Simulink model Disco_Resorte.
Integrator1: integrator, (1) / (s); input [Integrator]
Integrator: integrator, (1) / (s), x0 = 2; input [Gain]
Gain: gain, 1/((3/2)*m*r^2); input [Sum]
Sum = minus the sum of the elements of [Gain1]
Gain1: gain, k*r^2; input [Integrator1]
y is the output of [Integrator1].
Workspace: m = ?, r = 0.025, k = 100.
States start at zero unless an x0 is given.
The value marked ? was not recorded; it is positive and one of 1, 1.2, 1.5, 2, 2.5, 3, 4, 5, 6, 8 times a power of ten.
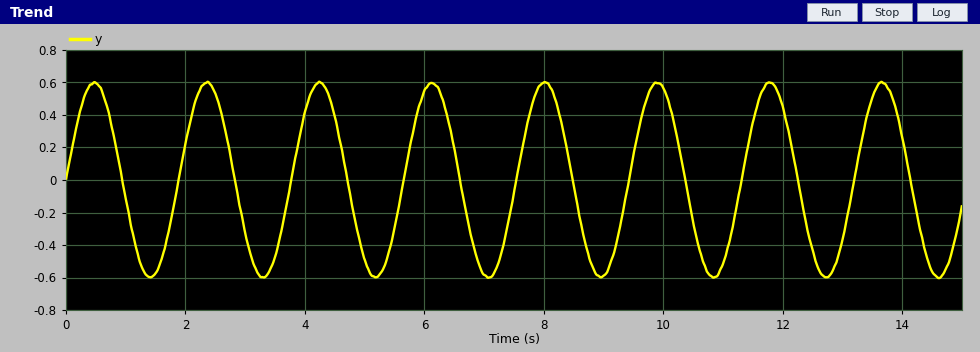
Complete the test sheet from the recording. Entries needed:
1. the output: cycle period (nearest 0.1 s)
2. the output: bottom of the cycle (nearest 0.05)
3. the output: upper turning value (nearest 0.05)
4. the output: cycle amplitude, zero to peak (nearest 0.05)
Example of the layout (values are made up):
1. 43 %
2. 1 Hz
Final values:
1. 1.9 s
2. -0.60
3. 0.60
4. 0.60
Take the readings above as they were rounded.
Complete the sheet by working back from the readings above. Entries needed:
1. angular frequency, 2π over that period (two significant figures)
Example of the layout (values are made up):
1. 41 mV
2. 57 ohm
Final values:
1. 3.3 rad/s
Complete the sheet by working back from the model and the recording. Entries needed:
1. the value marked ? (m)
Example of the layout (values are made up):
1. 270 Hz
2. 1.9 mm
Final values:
1. 6
